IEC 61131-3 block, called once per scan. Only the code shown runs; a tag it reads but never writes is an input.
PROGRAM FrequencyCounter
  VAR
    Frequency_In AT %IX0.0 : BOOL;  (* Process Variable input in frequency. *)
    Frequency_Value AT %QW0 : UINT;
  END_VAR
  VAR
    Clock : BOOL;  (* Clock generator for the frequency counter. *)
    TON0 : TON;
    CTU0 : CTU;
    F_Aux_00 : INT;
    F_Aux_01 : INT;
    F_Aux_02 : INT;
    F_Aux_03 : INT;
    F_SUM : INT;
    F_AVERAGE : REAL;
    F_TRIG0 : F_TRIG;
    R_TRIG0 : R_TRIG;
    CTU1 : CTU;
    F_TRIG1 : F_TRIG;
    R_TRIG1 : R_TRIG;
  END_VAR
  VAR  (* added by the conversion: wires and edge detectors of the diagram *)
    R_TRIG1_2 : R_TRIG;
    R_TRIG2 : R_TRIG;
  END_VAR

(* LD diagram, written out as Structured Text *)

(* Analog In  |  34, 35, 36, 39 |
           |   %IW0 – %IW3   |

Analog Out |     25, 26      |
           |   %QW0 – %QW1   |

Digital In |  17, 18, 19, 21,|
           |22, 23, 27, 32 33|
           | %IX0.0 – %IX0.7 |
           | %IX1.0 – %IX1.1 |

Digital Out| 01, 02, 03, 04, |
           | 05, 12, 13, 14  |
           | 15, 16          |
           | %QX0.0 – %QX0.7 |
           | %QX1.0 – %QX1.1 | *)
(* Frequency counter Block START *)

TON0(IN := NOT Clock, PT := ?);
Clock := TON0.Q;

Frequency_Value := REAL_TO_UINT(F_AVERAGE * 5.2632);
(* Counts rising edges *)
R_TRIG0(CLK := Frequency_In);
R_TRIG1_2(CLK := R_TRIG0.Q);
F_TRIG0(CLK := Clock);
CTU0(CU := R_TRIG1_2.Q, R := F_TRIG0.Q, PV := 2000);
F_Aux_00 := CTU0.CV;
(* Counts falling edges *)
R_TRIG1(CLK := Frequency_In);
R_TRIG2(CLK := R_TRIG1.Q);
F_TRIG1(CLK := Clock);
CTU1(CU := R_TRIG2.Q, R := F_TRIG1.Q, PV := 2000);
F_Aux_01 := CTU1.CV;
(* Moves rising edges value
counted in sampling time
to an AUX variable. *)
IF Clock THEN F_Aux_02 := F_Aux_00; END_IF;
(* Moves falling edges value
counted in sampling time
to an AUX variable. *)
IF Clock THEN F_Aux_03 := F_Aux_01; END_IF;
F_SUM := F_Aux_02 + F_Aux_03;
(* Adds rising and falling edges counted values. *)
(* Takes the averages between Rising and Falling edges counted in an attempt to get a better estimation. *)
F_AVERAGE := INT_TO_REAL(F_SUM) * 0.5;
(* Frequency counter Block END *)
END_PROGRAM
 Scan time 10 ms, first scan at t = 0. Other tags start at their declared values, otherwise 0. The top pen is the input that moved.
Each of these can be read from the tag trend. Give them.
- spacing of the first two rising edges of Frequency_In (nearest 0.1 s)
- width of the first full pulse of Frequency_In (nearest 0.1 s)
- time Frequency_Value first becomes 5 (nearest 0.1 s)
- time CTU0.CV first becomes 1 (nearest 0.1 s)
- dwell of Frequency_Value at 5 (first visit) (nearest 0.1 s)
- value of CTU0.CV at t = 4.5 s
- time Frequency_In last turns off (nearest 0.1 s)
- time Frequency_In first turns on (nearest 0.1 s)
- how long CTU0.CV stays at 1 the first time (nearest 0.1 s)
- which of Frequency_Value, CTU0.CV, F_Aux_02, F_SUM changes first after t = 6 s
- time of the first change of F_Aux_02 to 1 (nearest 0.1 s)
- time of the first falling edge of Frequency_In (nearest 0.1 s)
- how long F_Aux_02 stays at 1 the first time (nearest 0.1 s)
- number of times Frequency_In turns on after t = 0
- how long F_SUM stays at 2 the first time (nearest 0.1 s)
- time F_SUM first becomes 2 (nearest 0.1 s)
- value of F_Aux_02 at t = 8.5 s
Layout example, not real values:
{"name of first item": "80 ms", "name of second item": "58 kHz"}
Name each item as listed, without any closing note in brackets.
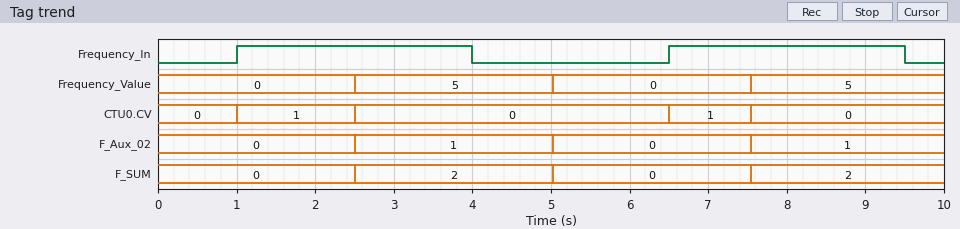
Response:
{"spacing of the first two rising edges of Frequency_In": "5.5 s", "width of the first full pulse of Frequency_In": "3.0 s", "time Frequency_Value first becomes 5": "2.5 s", "time CTU0.CV first becomes 1": "1.0 s", "dwell of Frequency_Value at 5 (first visit)": "2.5 s", "value of CTU0.CV at t = 4.5 s": "0", "time Frequency_In last turns off": "9.5 s", "time Frequency_In first turns on": "1.0 s", "how long CTU0.CV stays at 1 the first time": "1.5 s", "which of Frequency_Value, CTU0.CV, F_Aux_02, F_SUM changes first after t = 6 s": "CTU0.CV", "time of the first change of F_Aux_02 to 1": "2.5 s", "time of the first falling edge of Frequency_In": "4.0 s", "how long F_Aux_02 stays at 1 the first time": "2.5 s", "number of times Frequency_In turns on after t = 0": "2", "how long F_SUM stays at 2 the first time": "2.5 s", "time F_SUM first becomes 2": "2.5 s", "value of F_Aux_02 at t = 8.5 s": "1"}
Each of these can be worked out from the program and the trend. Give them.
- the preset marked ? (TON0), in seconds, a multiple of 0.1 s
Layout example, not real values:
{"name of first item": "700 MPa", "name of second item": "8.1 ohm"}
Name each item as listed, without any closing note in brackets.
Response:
{"the preset marked ? (TON0), in seconds, a multiple of 0.1 s": "2.5 s"}
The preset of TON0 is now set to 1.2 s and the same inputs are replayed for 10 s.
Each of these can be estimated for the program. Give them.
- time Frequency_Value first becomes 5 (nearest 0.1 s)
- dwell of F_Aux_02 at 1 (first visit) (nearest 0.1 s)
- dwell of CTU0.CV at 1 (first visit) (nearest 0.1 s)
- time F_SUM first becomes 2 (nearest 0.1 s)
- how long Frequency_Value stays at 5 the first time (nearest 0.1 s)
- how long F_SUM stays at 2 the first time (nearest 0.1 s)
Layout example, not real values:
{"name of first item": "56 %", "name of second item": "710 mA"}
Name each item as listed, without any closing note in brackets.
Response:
{"time Frequency_Value first becomes 5": "1.2 s", "dwell of F_Aux_02 at 1 (first visit)": "1.2 s", "dwell of CTU0.CV at 1 (first visit)": "0.2 s", "time F_SUM first becomes 2": "1.2 s", "how long Frequency_Value stays at 5 the first time": "1.2 s", "how long F_SUM stays at 2 the first time": "1.2 s"}
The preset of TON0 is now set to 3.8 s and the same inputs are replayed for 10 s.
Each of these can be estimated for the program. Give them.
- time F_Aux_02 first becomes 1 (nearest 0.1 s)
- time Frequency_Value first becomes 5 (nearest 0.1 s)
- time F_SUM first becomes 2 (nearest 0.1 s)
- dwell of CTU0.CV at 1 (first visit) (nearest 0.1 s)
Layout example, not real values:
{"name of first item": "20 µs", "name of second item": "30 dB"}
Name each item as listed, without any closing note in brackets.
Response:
{"time F_Aux_02 first becomes 1": "3.8 s", "time Frequency_Value first becomes 5": "3.8 s", "time F_SUM first becomes 2": "3.8 s", "dwell of CTU0.CV at 1 (first visit)": "2.8 s"}
